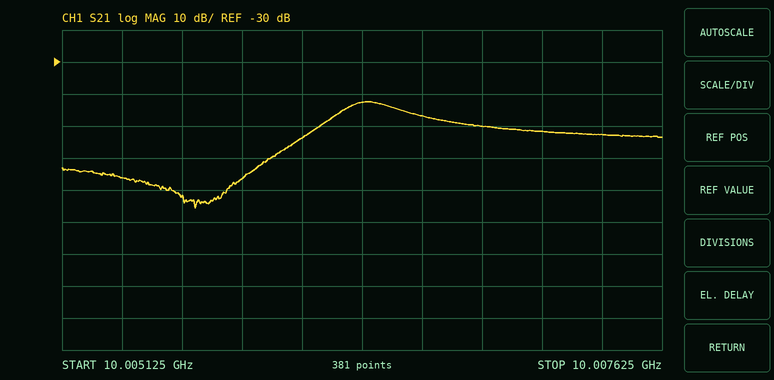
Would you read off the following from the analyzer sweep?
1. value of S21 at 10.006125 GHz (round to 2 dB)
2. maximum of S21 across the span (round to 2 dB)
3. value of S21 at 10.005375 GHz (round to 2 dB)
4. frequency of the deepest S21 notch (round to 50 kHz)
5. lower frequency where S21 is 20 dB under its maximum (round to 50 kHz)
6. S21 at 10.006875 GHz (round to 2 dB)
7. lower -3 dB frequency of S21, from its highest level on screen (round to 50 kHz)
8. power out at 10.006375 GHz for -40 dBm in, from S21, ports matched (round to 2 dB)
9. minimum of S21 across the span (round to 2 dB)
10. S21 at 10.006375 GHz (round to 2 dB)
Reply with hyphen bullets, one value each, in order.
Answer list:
- -54 dB
- -42 dB
- -66 dB
- 10.00570 GHz
- 10.00595 GHz
- -50 dB
- 10.00630 GHz
- -82 dBm
- -76 dB
- -42 dB
